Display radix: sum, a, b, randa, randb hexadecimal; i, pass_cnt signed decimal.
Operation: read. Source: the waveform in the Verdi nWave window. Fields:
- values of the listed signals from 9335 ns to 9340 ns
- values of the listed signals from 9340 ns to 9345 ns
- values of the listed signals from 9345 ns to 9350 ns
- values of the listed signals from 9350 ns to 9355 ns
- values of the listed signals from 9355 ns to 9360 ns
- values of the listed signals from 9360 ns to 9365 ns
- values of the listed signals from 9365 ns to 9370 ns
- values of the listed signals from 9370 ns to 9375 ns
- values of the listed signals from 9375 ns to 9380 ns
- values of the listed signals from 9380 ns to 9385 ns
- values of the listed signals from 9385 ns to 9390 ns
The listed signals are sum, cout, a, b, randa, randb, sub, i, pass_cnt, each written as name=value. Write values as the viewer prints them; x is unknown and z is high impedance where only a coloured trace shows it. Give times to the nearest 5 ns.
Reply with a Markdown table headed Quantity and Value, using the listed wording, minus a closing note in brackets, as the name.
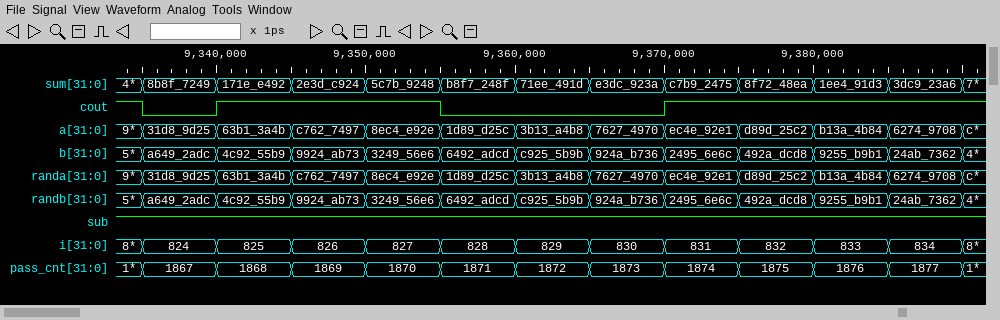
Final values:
| Quantity | Value |
|---|---|
| values of the listed signals from 9335 ns to 9340 ns | sum=8b8f_7249, cout=0, a=31d8_9d25, b=a649_2adc, randa=31d8_9d25, randb=a649_2adc, sub=1, i=824, pass_cnt=1867 |
| values of the listed signals from 9340 ns to 9345 ns | sum=171e_e492, cout=1, a=63b1_3a4b, b=4c92_55b9, randa=63b1_3a4b, randb=4c92_55b9, sub=1, i=825, pass_cnt=1868 |
| values of the listed signals from 9345 ns to 9350 ns | sum=2e3d_c924, cout=1, a=c762_7497, b=9924_ab73, randa=c762_7497, randb=9924_ab73, sub=1, i=826, pass_cnt=1869 |
| values of the listed signals from 9350 ns to 9355 ns | sum=5c7b_9248, cout=1, a=8ec4_e92e, b=3249_56e6, randa=8ec4_e92e, randb=3249_56e6, sub=1, i=827, pass_cnt=1870 |
| values of the listed signals from 9355 ns to 9360 ns | sum=b8f7_248f, cout=0, a=1d89_d25c, b=6492_adcd, randa=1d89_d25c, randb=6492_adcd, sub=1, i=828, pass_cnt=1871 |
| values of the listed signals from 9360 ns to 9365 ns | sum=71ee_491d, cout=0, a=3b13_a4b8, b=c925_5b9b, randa=3b13_a4b8, randb=c925_5b9b, sub=1, i=829, pass_cnt=1872 |
| values of the listed signals from 9365 ns to 9370 ns | sum=e3dc_923a, cout=0, a=7627_4970, b=924a_b736, randa=7627_4970, randb=924a_b736, sub=1, i=830, pass_cnt=1873 |
| values of the listed signals from 9370 ns to 9375 ns | sum=c7b9_2475, cout=1, a=ec4e_92e1, b=2495_6e6c, randa=ec4e_92e1, randb=2495_6e6c, sub=1, i=831, pass_cnt=1874 |
| values of the listed signals from 9375 ns to 9380 ns | sum=8f72_48ea, cout=1, a=d89d_25c2, b=492a_dcd8, randa=d89d_25c2, randb=492a_dcd8, sub=1, i=832, pass_cnt=1875 |
| values of the listed signals from 9380 ns to 9385 ns | sum=1ee4_91d3, cout=1, a=b13a_4b84, b=9255_b9b1, randa=b13a_4b84, randb=9255_b9b1, sub=1, i=833, pass_cnt=1876 |
| values of the listed signals from 9385 ns to 9390 ns | sum=3dc9_23a6, cout=1, a=6274_9708, b=24ab_7362, randa=6274_9708, randb=24ab_7362, sub=1, i=834, pass_cnt=1877 |
